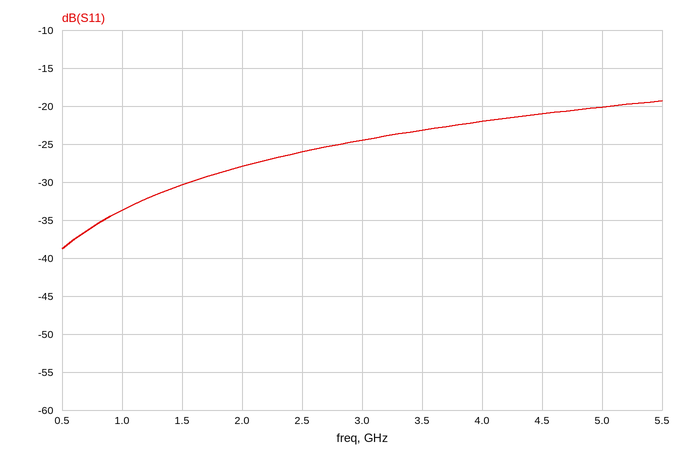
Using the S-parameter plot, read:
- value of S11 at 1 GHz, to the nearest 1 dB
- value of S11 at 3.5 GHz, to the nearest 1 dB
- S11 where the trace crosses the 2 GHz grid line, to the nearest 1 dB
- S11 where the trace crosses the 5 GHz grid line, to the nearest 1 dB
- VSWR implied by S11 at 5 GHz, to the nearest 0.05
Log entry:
-34 dB
-23 dB
-28 dB
-20 dB
1.20
